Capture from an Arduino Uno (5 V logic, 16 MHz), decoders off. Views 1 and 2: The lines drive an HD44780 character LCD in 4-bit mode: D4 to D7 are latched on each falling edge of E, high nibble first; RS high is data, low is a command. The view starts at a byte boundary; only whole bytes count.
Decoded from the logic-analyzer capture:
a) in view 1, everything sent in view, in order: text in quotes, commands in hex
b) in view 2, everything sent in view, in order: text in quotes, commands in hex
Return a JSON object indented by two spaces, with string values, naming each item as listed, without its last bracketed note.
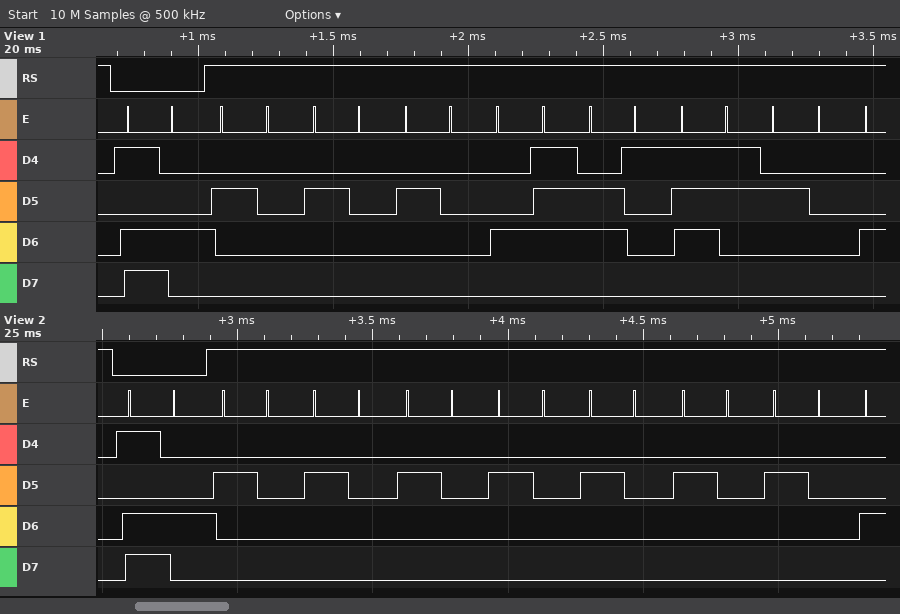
{
  "in view 1, everything sent in view, in order: text in quotes, commands in hex": "0xD4 \"   Gas \"",
  "in view 2, everything sent in view, in order: text in quotes, commands in hex": "0xD4 \"       \""
}
